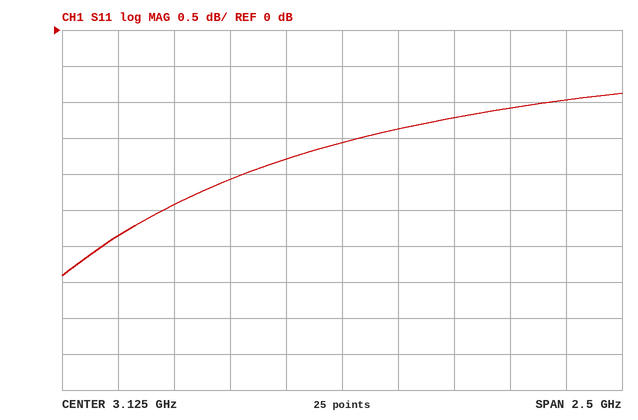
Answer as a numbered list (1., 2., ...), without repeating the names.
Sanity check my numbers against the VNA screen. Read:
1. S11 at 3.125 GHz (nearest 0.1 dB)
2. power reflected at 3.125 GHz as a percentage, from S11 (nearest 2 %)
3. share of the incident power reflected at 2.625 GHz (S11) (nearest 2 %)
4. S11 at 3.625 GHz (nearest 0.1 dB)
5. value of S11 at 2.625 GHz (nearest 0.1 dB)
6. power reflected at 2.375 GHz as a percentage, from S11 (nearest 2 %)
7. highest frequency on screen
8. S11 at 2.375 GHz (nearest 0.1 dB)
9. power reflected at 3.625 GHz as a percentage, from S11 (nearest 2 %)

1. -1.6 dB
2. 70 %
3. 62 %
4. -1.2 dB
5. -2.1 dB
6. 58 %
7. 4.375 GHz
8. -2.4 dB
9. 76 %
